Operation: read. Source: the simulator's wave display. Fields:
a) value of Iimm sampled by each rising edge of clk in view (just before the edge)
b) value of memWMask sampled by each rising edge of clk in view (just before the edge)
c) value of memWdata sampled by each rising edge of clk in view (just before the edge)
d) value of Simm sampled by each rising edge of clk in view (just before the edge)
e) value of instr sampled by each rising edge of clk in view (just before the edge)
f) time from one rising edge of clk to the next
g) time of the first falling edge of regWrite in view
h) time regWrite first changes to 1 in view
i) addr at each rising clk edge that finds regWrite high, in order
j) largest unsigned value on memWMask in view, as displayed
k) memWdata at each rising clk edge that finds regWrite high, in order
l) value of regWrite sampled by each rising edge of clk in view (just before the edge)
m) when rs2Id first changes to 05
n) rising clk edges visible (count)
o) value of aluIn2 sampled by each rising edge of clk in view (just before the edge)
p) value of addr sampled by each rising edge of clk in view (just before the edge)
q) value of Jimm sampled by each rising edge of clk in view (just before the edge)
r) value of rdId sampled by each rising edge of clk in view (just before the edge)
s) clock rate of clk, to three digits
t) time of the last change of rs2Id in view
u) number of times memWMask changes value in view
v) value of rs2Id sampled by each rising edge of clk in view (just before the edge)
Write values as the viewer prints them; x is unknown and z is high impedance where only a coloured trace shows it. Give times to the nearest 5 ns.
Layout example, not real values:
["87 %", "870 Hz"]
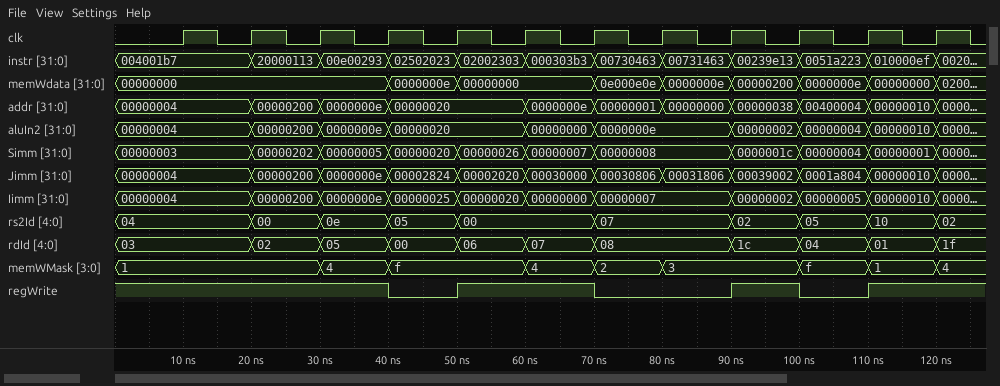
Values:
["00000004, 00000004, 00000200, 0000000e, 00000025, 00000020, 00000000, 00000007, 00000007, 00000002, 00000005, 00000010", "1, 1, 1, 4, f, f, 4, 2, 3, 3, f, 1", "00000000, 00000000, 00000000, 00000000, 0000000e, 00000000, 00000000, 0e000e0e, 0000000e, 00000200, 0000000e, 00000000", "00000003, 00000003, 00000202, 00000005, 00000020, 00000026, 00000007, 00000008, 00000008, 0000001c, 00000004, 00000001", "004001b7, 004001b7, 20000113, 00e00293, 02502023, 02002303, 000303b3, 00730463, 00731463, 00239e13, 0051a223, 010000ef", "10 ns", "40 ns", "50 ns", "00000004, 00000004, 00000200, 0000000e, 00000020, 0000000e, 00000038, 00000010", "f", "00000000, 00000000, 00000000, 00000000, 00000000, 00000000, 00000200, 00000000", "1 1 1 1 0 1 1 0 0 1 0 1", "40 ns", "12", "00000004, 00000004, 00000200, 0000000e, 00000020, 00000020, 00000000, 0000000e, 0000000e, 00000002, 00000004, 00000010", "00000004, 00000004, 00000200, 0000000e, 00000020, 00000020, 0000000e, 00000001, 00000000, 00000038, 00400004, 00000010", "00000004, 00000004, 00000200, 0000000e, 00002824, 00002020, 00030000, 00030806, 00031806, 00039002, 0001a804, 00000010", "03, 03, 02, 05, 00, 06, 07, 08, 08, 1c, 04, 01", "100 MHz", "120 ns", "8", "04, 04, 00, 0e, 05, 00, 00, 07, 07, 02, 05, 10"]
